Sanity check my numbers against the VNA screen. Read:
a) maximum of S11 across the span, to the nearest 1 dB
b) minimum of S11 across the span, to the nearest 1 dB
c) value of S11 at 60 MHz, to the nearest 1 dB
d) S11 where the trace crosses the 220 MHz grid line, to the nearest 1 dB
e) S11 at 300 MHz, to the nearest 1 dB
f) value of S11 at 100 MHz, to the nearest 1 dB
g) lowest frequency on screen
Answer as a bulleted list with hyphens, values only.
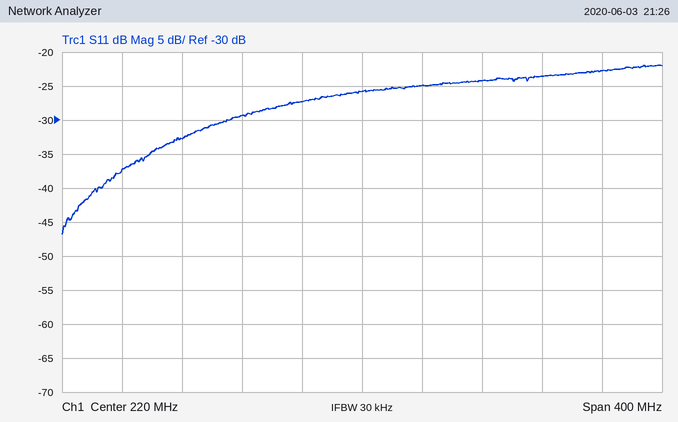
- -22 dB
- -47 dB
- -37 dB
- -26 dB
- -24 dB
- -33 dB
- 20 MHz
